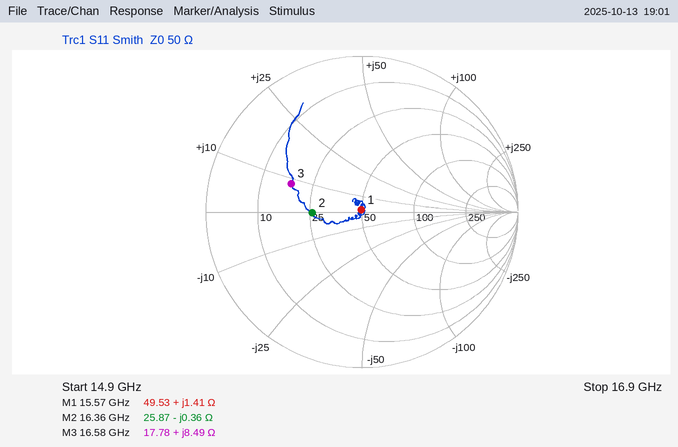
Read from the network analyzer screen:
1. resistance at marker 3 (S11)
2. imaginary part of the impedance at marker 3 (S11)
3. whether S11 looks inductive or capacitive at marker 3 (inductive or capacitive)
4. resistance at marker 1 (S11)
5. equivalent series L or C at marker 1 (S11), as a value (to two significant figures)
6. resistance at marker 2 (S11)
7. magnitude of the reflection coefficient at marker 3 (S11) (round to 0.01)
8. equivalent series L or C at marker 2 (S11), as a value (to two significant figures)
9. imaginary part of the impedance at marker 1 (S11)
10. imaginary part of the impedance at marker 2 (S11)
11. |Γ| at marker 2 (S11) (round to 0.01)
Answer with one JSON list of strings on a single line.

["17.78 Ω", "+8.49 Ω", "inductive", "49.53 Ω", "14 pH", "25.87 Ω", "0.49", "27 pF", "+1.41 Ω", "-0.36 Ω", "0.32"]
